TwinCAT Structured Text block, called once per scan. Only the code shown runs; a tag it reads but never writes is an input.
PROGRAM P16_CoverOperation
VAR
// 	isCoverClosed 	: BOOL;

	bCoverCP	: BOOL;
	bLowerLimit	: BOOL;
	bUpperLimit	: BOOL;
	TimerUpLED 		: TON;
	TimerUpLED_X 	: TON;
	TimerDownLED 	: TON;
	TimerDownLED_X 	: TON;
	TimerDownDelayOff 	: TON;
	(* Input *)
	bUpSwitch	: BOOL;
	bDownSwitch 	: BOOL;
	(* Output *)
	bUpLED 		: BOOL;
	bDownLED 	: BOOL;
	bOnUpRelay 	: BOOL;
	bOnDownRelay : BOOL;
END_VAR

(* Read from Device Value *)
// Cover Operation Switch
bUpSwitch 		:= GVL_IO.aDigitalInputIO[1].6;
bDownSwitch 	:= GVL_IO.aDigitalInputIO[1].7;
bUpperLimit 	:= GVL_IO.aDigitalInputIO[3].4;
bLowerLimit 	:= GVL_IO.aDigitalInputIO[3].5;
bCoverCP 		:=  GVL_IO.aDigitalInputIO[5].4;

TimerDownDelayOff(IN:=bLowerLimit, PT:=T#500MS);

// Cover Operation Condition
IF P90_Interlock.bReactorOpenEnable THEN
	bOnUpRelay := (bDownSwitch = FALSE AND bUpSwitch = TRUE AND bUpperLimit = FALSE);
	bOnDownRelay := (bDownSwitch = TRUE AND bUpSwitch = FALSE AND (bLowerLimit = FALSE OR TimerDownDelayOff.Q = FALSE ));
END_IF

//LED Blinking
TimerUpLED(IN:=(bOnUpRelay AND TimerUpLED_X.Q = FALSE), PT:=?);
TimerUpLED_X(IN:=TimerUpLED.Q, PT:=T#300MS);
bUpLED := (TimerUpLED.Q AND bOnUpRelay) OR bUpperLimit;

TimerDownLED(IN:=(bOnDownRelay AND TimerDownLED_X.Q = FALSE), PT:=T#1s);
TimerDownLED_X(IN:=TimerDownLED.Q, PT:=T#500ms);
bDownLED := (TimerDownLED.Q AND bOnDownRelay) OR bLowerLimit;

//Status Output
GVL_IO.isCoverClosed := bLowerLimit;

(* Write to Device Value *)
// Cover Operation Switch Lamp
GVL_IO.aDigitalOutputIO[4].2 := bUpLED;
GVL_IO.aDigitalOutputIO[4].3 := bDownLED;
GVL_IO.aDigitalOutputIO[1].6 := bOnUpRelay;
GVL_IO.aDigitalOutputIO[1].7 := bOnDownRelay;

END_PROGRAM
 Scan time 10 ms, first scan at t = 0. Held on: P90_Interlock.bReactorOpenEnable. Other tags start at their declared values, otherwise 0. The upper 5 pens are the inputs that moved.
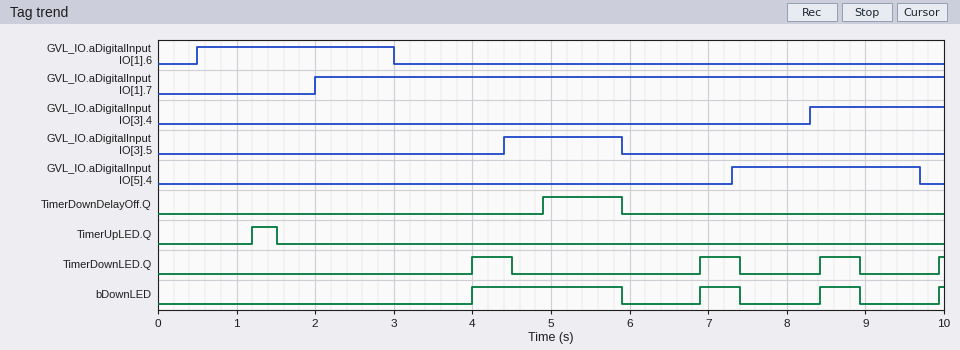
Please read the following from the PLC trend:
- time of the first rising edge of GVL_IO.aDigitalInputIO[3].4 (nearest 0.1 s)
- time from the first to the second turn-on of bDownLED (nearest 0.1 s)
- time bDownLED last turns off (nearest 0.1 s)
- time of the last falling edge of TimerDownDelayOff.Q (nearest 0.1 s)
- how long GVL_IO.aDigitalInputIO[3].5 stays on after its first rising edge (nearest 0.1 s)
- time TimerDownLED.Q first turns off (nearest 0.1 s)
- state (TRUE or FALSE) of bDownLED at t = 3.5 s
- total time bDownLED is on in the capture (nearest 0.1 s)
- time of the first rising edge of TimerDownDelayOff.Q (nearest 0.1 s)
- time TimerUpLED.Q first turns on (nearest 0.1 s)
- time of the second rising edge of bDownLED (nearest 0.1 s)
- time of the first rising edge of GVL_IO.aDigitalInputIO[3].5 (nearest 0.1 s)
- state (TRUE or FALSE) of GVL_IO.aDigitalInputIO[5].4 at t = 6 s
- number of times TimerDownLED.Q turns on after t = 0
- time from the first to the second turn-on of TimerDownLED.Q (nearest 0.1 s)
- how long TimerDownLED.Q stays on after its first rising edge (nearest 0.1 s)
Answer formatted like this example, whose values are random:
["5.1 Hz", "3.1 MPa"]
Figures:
["8.3 s", "2.9 s", "8.9 s", "5.9 s", "1.5 s", "4.5 s", "FALSE", "3.0 s", "4.9 s", "1.2 s", "6.9 s", "4.4 s", "FALSE", "4", "2.9 s", "0.5 s"]
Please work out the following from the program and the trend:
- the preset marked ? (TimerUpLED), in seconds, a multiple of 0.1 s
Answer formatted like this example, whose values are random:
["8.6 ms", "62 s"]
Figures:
["0.7 s"]
